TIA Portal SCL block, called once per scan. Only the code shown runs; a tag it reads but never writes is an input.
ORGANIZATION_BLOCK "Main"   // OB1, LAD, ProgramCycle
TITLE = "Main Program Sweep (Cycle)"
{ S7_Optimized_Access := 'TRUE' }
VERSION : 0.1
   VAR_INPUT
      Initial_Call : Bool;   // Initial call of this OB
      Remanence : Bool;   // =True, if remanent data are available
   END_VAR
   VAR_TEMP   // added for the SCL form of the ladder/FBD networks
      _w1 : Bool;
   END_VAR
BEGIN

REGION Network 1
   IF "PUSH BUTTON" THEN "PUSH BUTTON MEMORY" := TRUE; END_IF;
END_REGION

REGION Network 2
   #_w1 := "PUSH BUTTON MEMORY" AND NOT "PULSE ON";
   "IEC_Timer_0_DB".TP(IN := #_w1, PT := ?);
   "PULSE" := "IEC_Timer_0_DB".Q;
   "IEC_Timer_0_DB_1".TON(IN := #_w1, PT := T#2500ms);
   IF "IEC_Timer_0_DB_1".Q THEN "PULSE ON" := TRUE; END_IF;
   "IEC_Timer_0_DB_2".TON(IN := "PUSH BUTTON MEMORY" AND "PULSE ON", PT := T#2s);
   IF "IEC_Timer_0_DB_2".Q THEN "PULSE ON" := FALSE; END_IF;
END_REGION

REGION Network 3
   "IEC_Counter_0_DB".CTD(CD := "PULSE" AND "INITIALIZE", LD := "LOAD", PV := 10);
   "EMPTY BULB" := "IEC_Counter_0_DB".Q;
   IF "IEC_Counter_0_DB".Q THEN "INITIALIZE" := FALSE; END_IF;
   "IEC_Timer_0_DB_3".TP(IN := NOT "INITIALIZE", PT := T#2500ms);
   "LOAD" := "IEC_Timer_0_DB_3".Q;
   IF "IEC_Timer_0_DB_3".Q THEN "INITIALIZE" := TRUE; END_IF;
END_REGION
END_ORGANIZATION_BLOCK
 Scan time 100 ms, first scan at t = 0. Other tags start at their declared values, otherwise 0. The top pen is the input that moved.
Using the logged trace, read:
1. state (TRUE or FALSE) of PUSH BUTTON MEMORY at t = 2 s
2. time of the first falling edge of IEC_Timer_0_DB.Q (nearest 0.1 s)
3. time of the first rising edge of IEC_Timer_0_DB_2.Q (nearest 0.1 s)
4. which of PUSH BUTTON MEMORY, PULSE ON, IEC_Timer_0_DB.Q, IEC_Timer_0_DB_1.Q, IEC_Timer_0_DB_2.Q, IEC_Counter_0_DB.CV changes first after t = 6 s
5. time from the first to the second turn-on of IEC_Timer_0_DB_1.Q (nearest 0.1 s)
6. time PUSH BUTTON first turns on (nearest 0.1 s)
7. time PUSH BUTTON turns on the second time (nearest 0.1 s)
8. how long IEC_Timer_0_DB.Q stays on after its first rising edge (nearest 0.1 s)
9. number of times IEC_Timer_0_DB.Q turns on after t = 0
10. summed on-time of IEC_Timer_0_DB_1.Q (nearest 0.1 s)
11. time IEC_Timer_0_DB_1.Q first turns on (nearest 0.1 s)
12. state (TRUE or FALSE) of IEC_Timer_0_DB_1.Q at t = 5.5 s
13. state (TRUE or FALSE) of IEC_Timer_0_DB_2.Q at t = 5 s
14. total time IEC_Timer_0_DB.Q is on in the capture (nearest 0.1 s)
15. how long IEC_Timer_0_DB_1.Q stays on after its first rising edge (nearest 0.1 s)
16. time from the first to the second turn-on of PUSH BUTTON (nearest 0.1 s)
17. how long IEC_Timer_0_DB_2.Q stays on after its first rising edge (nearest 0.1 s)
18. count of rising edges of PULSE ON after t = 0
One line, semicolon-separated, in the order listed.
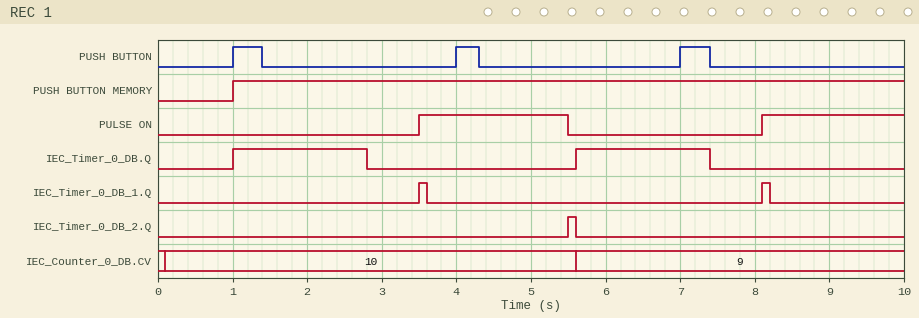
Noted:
TRUE; 2.8 s; 5.5 s; IEC_Timer_0_DB.Q; 4.6 s; 1.0 s; 4.0 s; 1.8 s; 2; 0.2 s; 3.5 s; FALSE; FALSE; 3.6 s; 0.1 s; 3.0 s; 0.1 s; 2
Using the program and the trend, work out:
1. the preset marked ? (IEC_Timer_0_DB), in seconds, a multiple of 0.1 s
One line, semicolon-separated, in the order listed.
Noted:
1.8 s
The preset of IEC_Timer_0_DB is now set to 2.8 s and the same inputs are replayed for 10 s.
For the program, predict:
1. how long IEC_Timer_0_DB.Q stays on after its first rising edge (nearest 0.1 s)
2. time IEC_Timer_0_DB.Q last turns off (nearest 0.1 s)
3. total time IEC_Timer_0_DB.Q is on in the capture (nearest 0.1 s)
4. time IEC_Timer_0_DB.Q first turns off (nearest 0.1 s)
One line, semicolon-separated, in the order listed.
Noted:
2.8 s; 8.4 s; 5.6 s; 3.8 s
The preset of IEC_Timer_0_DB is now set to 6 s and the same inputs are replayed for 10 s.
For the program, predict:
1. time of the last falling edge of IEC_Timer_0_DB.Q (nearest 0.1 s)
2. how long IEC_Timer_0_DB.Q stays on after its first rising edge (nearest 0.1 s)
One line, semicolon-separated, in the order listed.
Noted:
7.0 s; 6.0 s
